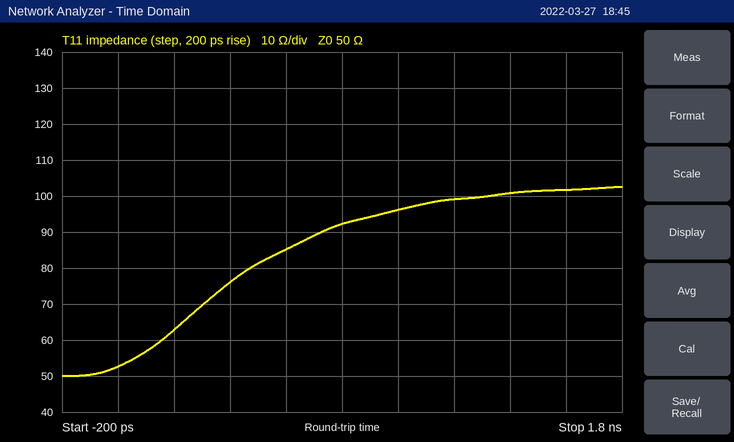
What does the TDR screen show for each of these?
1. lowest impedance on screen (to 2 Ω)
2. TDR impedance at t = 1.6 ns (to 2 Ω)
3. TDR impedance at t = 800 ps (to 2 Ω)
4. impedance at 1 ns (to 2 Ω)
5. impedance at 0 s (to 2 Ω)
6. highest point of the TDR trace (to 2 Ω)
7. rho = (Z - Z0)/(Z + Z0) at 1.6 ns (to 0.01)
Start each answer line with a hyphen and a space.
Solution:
- 50 Ω
- 102 Ω
- 92 Ω
- 96 Ω
- 52 Ω
- 102 Ω
- +0.34
